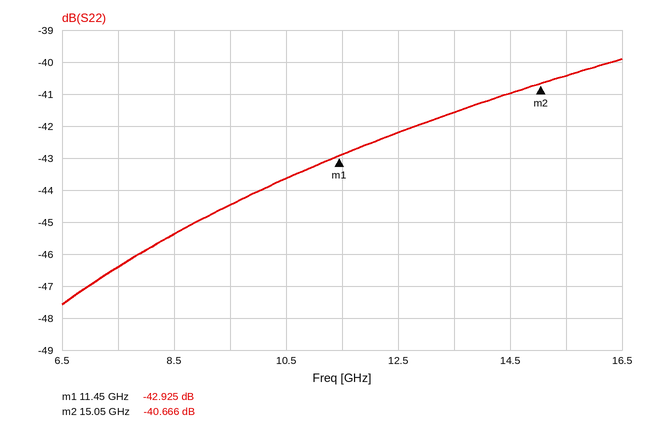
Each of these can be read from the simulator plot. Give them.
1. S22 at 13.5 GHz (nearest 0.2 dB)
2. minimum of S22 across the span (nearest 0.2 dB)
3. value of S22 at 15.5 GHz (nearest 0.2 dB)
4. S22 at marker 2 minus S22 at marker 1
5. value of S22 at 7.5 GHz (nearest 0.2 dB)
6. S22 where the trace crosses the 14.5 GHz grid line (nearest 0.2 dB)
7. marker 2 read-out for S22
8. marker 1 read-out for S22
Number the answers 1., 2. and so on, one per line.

1. -41.6 dB
2. -47.6 dB
3. -40.4 dB
4. 2.259 dB
5. -46.4 dB
6. -41.0 dB
7. -40.666 dB
8. -42.925 dB
